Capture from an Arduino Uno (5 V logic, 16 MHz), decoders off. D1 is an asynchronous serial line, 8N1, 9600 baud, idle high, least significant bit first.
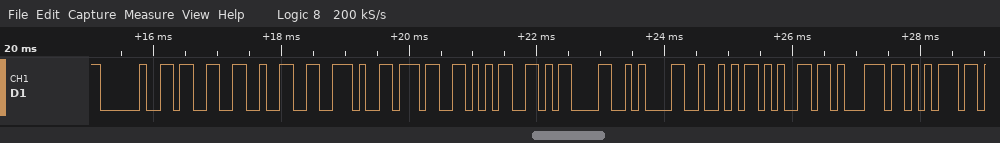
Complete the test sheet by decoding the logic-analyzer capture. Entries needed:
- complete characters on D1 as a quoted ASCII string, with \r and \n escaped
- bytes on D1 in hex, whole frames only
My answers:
" 32.75\r\nRequ"
20 33 32 2E 37 35 0D 0A 52 65 71 75
